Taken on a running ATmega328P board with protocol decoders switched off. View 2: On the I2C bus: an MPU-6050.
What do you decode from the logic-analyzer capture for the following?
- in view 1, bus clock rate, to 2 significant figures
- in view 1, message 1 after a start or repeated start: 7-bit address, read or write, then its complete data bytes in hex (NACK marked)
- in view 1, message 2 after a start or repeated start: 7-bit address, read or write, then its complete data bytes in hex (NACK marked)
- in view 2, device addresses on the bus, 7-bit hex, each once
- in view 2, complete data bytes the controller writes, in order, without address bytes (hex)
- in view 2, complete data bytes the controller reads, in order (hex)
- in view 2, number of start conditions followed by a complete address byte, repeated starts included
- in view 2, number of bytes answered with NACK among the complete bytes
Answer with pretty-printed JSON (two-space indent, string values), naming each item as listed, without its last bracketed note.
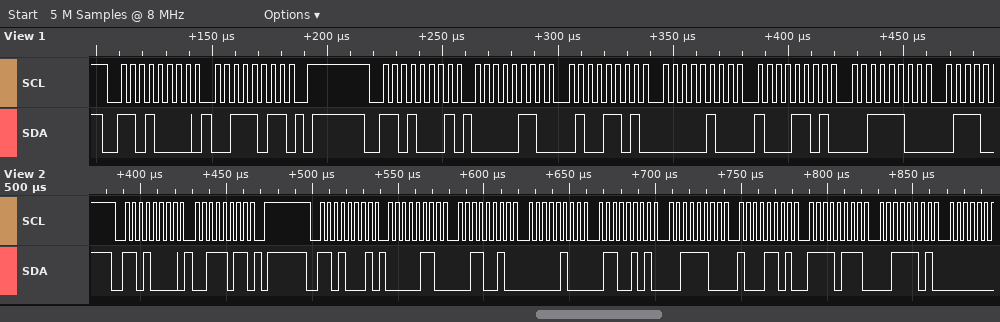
{
  "in view 1, bus clock rate, to 2 significant figures": "250 kHz",
  "in view 1, message 1 after a start or repeated start: 7-bit address, read or write, then its complete data bytes in hex": "0x68 write: 3B",
  "in view 1, message 2 after a start or repeated start: 7-bit address, read or write, then its complete data bytes in hex": "0x68 read: 06 4D 04 8D 3C",
  "in view 2, device addresses on the bus, 7-bit hex, each once": "0x68",
  "in view 2, complete data bytes the controller writes, in order, without address bytes": "3B",
  "in view 2, complete data bytes the controller reads, in order": "06 32 04 65 3C 8D F7 3D",
  "in view 2, number of start conditions followed by a complete address byte, repeated starts included": "2",
  "in view 2, number of bytes answered with NACK among the complete bytes": "0"
}
